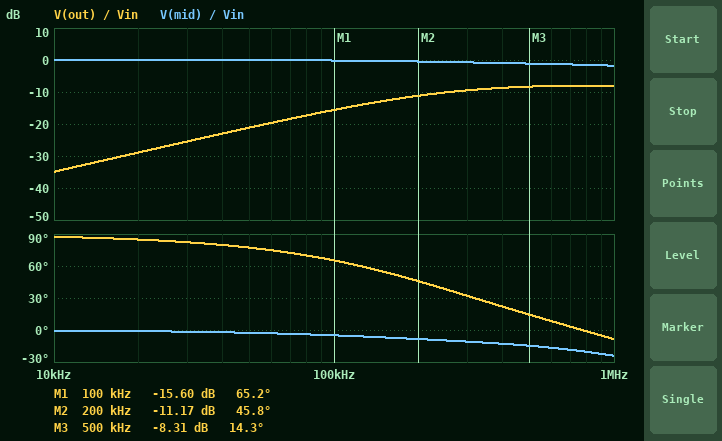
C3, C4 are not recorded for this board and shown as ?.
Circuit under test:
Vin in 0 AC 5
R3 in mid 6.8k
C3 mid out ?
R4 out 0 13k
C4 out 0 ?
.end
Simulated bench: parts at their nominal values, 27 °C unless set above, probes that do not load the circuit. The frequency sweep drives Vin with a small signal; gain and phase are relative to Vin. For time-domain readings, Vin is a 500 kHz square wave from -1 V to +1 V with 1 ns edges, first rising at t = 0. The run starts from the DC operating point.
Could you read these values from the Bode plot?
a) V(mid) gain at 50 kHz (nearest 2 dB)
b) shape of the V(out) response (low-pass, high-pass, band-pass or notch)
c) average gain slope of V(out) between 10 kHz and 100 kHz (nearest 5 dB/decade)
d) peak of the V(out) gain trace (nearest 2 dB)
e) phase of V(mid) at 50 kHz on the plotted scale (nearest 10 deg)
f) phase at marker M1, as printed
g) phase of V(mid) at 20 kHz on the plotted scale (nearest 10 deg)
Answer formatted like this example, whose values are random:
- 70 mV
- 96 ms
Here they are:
- 0 dB
- high-pass
- 20 dB/decade
- -8 dB
- 0 deg
- 65.2 deg
- 0 deg
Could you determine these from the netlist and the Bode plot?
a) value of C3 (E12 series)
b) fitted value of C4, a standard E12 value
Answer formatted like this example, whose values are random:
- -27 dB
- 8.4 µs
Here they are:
- 22 pF
- 22 pF
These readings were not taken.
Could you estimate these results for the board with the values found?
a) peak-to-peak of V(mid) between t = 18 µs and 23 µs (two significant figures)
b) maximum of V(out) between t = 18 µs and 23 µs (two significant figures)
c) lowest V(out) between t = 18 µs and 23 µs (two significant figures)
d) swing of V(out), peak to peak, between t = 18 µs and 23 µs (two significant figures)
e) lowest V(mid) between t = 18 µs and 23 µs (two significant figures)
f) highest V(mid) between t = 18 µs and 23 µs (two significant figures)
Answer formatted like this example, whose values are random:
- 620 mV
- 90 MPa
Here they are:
- 1.9 V
- 540 mV
- -540 mV
- 1.1 V
- -950 mV
- 950 mV
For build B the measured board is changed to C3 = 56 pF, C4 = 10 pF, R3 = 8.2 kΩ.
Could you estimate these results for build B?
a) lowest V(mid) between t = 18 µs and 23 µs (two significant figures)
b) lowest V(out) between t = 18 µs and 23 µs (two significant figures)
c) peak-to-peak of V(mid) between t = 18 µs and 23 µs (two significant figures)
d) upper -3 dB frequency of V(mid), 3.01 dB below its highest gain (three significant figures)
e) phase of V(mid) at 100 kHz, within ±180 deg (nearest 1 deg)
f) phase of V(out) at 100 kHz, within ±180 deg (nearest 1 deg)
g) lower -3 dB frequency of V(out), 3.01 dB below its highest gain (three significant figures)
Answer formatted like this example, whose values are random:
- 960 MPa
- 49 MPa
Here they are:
- -790 mV
- -680 mV
- 1.6 V
- 392 kHz
- -12 deg
- 50 deg
- 117 kHz
